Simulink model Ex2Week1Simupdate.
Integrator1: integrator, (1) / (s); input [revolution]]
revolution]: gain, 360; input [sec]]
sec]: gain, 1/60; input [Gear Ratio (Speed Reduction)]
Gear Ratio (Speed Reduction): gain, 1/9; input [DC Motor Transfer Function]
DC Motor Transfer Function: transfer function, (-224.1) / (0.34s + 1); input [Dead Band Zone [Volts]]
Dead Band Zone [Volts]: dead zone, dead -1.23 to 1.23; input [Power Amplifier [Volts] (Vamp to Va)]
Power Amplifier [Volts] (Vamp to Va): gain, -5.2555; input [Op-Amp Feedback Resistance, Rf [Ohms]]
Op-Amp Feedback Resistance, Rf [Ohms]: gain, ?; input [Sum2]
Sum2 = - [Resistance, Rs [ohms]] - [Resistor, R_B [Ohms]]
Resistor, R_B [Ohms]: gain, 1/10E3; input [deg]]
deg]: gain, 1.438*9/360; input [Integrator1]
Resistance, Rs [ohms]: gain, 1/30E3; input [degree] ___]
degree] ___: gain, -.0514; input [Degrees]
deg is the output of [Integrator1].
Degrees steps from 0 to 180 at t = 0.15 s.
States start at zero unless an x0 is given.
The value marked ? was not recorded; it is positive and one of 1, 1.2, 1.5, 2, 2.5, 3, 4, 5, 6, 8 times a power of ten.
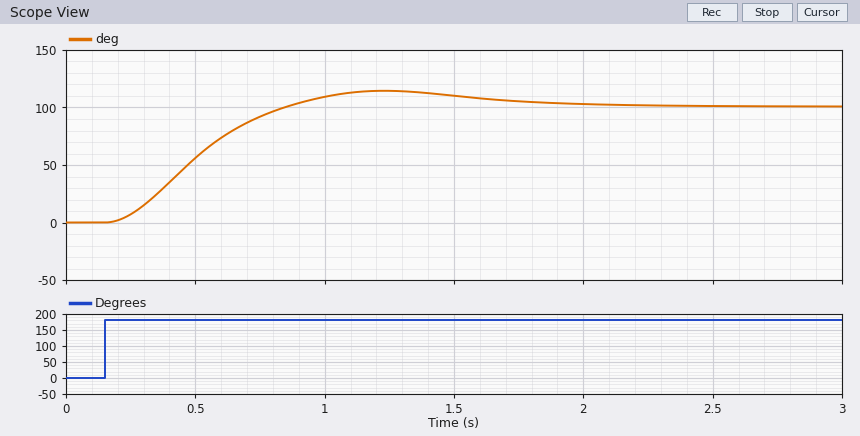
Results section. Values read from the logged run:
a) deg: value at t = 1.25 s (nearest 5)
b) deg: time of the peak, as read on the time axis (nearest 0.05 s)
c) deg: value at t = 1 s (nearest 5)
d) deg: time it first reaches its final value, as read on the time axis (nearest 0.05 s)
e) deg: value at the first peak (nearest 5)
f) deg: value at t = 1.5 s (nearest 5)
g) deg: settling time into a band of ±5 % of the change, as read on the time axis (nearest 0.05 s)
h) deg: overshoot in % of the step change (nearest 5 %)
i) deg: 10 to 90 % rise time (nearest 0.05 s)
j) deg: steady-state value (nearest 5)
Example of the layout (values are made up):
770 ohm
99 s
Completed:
115
1.25 s
110
0.85 s
115
110
1.70 s
15 %
0.45 s
100
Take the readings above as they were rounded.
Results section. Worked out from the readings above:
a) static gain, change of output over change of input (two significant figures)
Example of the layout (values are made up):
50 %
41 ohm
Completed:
0.56
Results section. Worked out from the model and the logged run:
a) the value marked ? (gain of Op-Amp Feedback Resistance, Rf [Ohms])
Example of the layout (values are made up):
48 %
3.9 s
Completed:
3000
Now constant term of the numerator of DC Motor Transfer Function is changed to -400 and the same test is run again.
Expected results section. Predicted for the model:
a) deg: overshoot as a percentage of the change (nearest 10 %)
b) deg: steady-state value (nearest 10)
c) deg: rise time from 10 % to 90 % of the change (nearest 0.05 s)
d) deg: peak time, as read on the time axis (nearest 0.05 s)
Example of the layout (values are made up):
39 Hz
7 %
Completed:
50 %
80
0.25 s
0.85 s
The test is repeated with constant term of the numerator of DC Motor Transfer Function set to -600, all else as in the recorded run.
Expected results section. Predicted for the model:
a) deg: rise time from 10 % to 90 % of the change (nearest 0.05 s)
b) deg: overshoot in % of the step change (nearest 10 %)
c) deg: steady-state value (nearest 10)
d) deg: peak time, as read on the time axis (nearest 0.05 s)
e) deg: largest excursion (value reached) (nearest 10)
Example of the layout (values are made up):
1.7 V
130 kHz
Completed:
0.15 s
100 %
70
0.70 s
130
